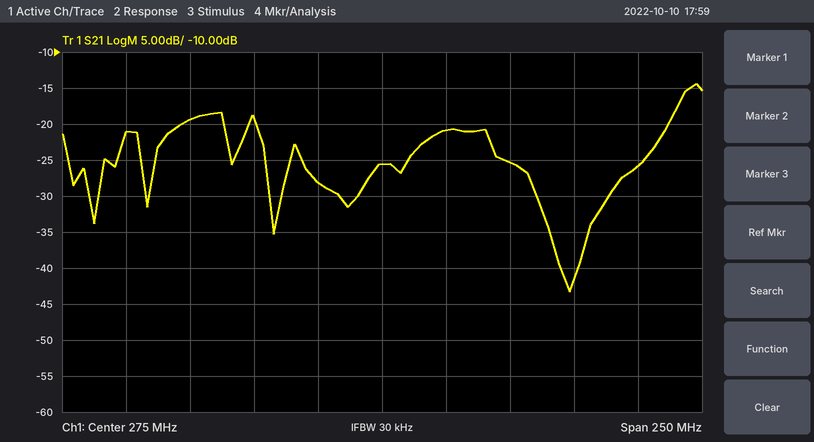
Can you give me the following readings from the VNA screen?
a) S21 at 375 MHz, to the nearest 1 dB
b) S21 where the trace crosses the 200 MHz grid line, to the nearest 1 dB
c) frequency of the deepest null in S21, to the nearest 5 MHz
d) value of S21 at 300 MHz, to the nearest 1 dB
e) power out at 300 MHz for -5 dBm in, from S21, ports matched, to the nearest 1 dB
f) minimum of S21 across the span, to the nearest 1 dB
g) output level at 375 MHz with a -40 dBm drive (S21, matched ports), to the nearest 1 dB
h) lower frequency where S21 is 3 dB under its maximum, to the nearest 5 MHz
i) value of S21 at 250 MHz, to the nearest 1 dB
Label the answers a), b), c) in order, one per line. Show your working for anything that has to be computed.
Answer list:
a) -26 dB
b) -19 dB
c) 350 MHz
d) -21 dB
e) -5 dBm + (-21 dB) = -26 dBm
f) -43 dB
g) -40 dBm + (-26 dB) = -66 dBm
h) 390 MHz
i) -28 dB
